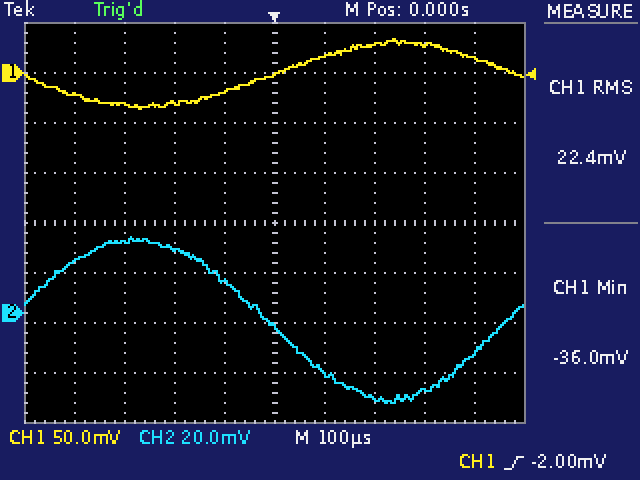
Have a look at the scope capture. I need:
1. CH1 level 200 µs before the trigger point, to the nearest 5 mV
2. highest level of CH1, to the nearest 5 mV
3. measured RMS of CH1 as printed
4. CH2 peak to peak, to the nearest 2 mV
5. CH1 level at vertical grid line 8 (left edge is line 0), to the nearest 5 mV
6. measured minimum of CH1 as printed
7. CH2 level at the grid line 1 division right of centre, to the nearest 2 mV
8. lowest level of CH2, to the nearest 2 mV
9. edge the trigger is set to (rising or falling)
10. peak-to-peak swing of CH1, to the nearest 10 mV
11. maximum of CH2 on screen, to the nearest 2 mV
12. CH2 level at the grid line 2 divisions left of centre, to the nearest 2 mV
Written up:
-30 mV
35 mV
22.4 mV
66 mV
30 mV
-36.0 mV
-24 mV
-36 mV
rising
70 mV
30 mV
26 mV
